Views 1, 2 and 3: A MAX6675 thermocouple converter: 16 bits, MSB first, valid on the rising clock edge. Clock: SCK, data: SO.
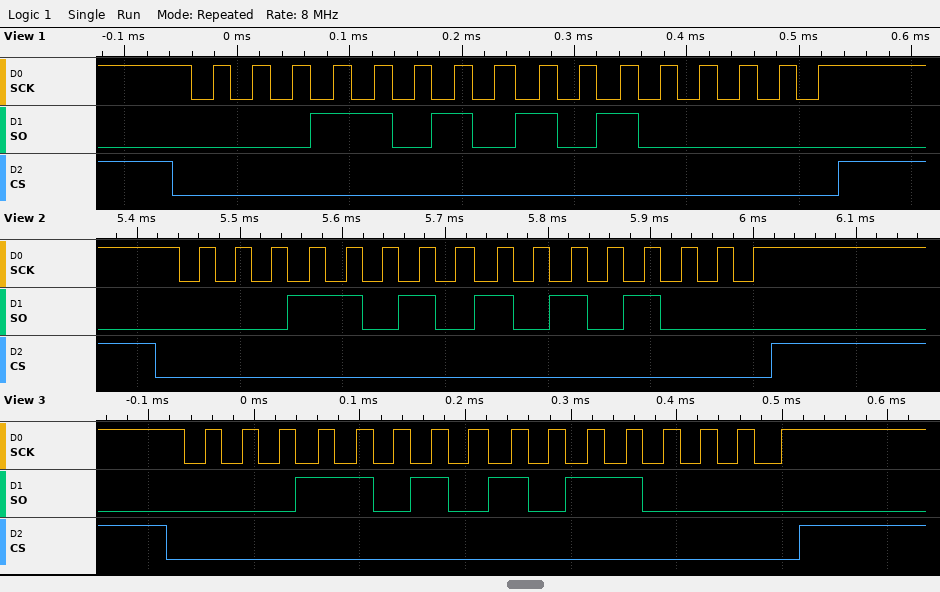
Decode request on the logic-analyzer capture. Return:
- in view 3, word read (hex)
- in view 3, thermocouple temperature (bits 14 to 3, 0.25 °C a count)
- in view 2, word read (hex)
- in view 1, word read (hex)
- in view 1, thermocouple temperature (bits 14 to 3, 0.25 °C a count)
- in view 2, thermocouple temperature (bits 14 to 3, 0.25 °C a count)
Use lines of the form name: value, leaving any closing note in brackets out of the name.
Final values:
in view 3, word read: 0x1AB0
in view 3, thermocouple temperature: 213.50 °C
in view 2, word read: 0x1AA8
in view 1, word read: 0x1AA0
in view 1, thermocouple temperature: 213.00 °C
in view 2, thermocouple temperature: 213.25 °C
